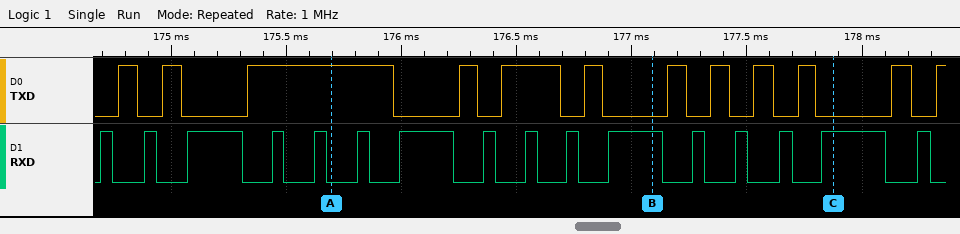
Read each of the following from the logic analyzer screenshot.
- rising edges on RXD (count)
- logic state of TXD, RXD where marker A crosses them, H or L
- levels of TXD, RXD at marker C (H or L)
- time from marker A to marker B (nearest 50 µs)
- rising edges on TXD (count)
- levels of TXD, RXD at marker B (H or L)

16
TXD=H, RXD=L
TXD=L, RXD=H
1400 µs
12
TXD=L, RXD=H
